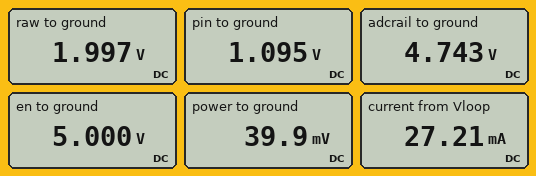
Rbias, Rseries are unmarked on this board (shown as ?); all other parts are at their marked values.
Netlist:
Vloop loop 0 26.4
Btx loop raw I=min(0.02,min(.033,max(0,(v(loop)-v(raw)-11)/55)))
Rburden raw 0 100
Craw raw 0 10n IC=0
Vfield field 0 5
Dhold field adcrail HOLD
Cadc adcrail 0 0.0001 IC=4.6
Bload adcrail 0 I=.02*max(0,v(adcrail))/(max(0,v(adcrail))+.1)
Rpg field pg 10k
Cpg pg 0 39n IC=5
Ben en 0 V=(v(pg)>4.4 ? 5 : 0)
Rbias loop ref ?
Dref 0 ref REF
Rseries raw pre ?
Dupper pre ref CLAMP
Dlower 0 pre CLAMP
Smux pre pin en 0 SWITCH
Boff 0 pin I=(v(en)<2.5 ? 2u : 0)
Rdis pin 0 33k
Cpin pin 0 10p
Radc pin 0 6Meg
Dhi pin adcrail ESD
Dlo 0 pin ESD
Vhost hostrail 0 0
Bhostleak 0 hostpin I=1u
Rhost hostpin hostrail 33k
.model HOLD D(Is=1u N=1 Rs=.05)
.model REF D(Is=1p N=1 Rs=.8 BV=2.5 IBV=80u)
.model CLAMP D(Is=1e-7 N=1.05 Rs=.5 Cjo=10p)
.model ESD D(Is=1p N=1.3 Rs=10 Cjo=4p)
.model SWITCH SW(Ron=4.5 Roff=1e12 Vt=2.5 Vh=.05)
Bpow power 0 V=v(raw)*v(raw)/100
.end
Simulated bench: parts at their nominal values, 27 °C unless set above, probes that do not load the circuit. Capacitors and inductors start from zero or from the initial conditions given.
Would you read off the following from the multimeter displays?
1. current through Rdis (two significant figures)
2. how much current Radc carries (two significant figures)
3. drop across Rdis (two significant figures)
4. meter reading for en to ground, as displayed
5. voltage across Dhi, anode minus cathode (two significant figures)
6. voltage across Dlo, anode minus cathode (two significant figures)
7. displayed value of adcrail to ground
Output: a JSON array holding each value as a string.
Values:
["33 µA", "180 nA", "1.1 V", "5.000 V", "-3.6 V", "-1.1 V", "4.743 V"]
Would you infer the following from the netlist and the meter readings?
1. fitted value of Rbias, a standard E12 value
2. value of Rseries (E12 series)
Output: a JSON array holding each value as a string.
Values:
["3.3 kΩ", "27 kΩ"]
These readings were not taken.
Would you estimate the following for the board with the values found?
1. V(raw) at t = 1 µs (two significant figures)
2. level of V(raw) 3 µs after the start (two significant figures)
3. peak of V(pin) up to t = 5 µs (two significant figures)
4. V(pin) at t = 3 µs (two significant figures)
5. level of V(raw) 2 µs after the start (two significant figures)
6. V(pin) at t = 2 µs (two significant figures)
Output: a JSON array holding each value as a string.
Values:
["1.3 V", "1.9 V", "1.1 V", "1.0 V", "1.7 V", "860 mV"]
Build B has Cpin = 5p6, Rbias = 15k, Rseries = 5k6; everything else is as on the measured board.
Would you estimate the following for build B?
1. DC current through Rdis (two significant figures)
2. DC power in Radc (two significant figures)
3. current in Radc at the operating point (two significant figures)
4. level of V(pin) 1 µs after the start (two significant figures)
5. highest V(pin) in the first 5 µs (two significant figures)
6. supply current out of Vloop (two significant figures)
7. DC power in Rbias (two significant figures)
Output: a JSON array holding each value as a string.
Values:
["52 µA", "480 nW", "280 nA", "1.0 V", "1.7 V", "22 mA", "38 mW"]
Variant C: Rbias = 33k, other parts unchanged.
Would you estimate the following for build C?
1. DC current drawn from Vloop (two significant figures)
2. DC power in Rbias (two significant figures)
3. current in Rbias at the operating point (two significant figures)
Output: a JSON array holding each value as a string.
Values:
["21 mA", "17 mW", "720 µA"]
